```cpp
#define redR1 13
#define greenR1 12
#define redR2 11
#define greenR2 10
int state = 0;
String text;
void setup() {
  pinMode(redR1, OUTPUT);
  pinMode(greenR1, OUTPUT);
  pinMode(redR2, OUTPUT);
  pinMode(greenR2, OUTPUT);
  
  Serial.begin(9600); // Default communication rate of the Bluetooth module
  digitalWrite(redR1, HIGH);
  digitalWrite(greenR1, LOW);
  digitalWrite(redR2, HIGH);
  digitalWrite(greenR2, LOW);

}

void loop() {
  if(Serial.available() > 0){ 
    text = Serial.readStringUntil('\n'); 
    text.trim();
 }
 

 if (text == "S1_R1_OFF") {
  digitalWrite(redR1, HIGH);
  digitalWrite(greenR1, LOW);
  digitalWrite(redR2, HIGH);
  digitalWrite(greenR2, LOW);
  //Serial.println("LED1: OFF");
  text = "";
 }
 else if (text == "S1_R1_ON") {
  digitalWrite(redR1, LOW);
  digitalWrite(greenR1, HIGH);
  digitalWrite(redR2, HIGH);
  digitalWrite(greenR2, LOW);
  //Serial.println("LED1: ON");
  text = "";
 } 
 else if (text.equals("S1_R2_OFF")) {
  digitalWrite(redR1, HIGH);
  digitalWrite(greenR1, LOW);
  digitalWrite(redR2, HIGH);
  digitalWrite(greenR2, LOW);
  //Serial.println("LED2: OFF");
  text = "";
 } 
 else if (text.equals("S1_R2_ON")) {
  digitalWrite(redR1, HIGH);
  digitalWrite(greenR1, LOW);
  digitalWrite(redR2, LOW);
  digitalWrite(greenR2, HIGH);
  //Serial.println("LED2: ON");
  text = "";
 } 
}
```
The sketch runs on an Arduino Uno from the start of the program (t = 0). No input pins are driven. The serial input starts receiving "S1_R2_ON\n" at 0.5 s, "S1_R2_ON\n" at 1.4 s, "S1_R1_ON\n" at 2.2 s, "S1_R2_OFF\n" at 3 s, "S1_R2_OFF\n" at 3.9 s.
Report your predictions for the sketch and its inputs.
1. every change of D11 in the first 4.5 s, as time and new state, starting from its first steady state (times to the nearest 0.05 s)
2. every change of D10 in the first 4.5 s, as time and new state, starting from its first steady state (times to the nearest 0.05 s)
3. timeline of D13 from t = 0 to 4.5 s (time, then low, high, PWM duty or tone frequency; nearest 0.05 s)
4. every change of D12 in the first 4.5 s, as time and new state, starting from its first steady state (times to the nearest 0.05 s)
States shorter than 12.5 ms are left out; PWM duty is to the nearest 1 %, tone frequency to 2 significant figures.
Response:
0 s high; 0.5 s low; 2.2 s high
0 s low; 0.5 s high; 2.2 s low
0 s high; 2.2 s low; 3 s high
0 s low; 2.2 s high; 3 s low
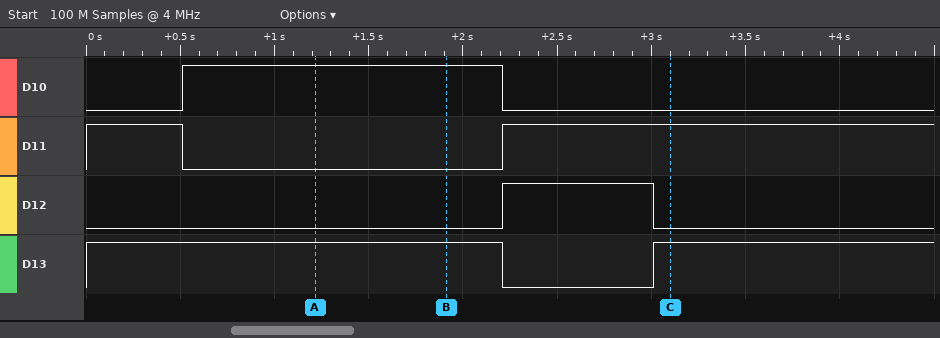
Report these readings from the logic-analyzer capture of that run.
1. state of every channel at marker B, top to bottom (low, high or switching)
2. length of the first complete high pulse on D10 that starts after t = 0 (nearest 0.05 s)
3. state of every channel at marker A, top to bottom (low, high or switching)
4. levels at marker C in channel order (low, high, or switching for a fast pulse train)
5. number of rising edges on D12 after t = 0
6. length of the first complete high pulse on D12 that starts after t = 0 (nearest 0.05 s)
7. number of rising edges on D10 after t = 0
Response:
D10 high, D11 low, D12 low, D13 high
1.70 s
D10 high, D11 low, D12 low, D13 high
D10 low, D11 high, D12 low, D13 high
1
0.80 s
1
